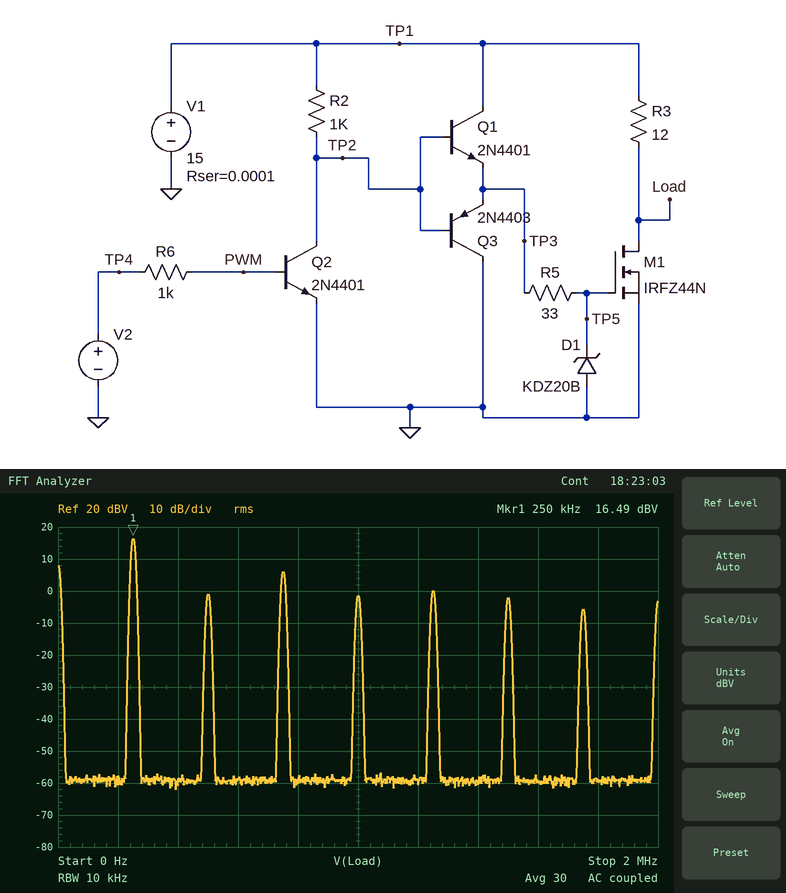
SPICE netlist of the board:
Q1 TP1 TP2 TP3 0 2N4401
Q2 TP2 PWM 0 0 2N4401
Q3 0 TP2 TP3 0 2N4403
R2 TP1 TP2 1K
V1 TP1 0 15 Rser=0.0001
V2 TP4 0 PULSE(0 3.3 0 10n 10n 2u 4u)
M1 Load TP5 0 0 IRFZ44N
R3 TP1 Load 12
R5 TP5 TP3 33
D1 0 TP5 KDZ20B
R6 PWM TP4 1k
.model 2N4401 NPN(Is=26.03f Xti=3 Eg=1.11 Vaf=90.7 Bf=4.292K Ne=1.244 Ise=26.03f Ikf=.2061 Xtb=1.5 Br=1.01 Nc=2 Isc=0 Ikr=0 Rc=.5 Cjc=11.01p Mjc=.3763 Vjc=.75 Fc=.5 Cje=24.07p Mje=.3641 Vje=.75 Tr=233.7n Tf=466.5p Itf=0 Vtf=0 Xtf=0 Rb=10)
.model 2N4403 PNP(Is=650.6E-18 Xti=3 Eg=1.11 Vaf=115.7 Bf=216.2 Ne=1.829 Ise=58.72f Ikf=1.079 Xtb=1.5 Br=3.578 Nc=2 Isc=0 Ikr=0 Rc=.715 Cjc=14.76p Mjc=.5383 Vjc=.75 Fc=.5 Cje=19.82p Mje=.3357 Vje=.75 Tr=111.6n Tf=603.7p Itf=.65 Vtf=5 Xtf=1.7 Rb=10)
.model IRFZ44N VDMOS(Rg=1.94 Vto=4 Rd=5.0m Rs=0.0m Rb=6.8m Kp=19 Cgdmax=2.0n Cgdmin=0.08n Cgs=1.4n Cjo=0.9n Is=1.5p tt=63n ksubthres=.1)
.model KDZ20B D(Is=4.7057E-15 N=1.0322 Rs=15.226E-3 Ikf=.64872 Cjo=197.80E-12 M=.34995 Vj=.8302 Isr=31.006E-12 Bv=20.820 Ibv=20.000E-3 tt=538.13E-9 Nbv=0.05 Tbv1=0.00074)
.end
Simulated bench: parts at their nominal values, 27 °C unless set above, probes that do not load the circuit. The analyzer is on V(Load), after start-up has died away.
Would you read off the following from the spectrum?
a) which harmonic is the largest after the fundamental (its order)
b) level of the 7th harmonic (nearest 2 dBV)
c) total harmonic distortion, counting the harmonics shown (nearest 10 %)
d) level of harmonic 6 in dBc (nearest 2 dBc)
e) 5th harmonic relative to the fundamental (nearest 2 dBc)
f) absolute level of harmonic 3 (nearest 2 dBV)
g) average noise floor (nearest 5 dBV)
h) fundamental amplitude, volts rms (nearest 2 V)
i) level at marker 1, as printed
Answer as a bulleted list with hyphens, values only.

- 3
- -6 dBV
- 40 %
- -18 dBc
- -16 dBc
- 6 dBV
- -60 dBV
- 6 V
- 16.49 dBV
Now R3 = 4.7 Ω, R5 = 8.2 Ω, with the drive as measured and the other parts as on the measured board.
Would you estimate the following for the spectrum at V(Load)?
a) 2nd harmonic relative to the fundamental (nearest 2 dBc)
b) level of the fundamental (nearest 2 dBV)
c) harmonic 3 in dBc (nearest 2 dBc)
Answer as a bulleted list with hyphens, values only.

- -12 dBc
- 16 dBV
- -12 dBc
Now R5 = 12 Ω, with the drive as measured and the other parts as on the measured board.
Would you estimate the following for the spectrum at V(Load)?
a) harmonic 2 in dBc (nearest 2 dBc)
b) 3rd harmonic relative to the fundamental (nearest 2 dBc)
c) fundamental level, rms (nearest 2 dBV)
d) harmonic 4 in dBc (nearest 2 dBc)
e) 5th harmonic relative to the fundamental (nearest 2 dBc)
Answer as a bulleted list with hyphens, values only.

- -12 dBc
- -12 dBc
- 16 dBV
- -14 dBc
- -22 dBc
